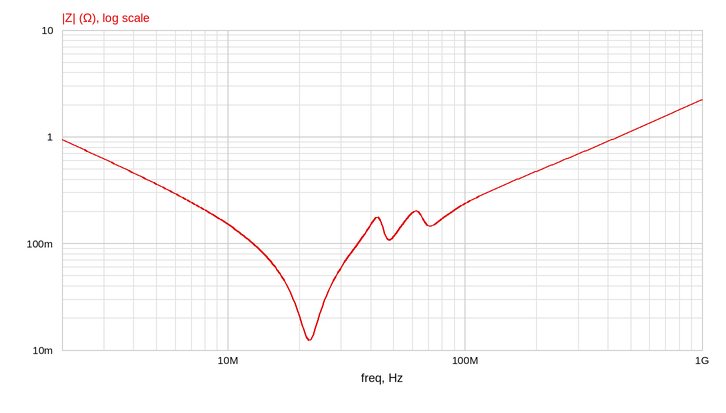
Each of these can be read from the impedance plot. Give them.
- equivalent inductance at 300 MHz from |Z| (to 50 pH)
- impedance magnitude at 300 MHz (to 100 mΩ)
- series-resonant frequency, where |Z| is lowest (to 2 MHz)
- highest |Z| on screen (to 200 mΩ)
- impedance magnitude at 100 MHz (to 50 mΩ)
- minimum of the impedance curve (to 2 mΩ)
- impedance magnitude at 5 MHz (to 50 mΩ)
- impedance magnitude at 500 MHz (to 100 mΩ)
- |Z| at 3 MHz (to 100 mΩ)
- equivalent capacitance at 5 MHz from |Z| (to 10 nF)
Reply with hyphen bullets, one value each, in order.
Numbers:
- 350 pH
- 700 mΩ
- 22 MHz
- 2.2 Ω
- 250 mΩ
- 12 mΩ
- 350 mΩ
- 1.1 Ω
- 600 mΩ
- 90 nF
